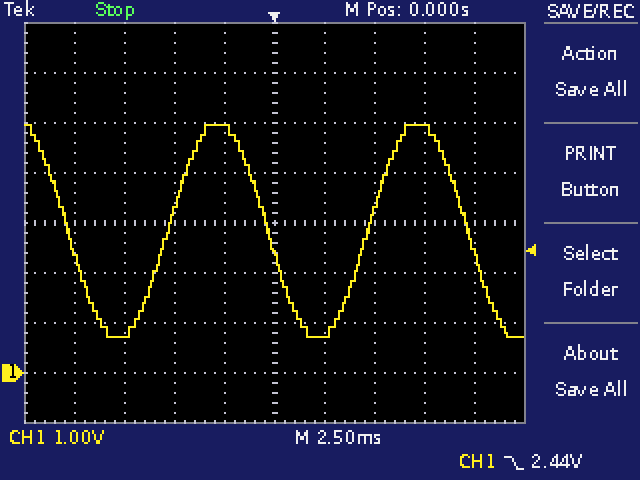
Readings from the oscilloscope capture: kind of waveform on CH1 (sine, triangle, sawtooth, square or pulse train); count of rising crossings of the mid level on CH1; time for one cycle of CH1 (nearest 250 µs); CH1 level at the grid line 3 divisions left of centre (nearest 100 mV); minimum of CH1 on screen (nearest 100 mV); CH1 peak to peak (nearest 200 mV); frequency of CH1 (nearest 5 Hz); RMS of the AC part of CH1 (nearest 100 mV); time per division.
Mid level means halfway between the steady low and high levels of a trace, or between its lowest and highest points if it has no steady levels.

sine
2
10.00 ms
700 mV
700 mV
4.2 V
100 Hz
1.5 V
2.5 ms
